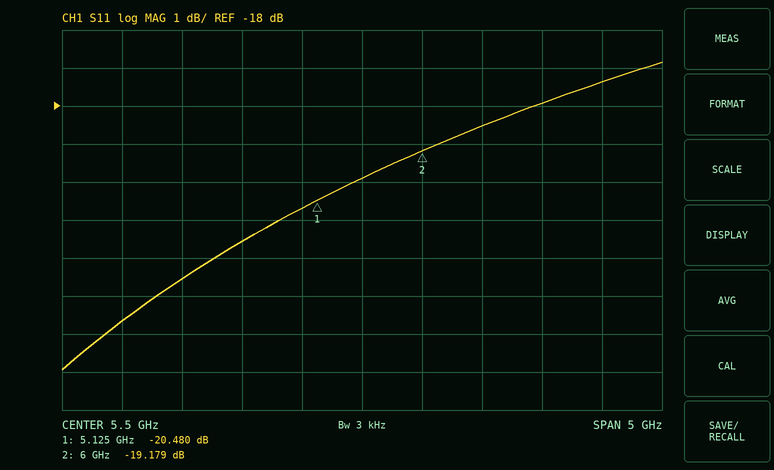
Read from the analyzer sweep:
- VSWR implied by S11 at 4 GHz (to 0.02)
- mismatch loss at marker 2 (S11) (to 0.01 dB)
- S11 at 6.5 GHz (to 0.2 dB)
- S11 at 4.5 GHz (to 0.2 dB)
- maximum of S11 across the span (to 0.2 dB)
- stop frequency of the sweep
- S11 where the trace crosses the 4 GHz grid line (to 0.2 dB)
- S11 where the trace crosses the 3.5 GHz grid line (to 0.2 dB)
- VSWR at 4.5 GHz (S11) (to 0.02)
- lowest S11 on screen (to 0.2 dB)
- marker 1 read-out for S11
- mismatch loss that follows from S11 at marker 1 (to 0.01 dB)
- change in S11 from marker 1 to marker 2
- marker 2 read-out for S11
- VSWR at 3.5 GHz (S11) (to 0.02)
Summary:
1.16
0.05 dB
-18.6 dB
-21.6 dB
-16.8 dB
8 GHz
-22.6 dB
-23.6 dB
1.18
-25.0 dB
-20.480 dB
0.04 dB
1.301 dB
-19.179 dB
1.14
